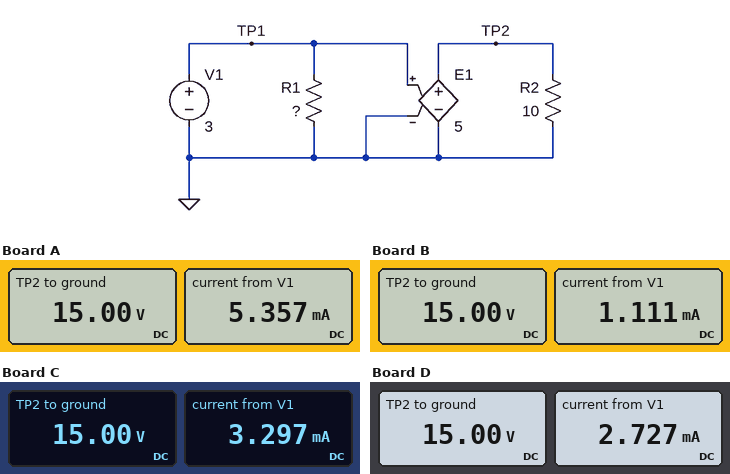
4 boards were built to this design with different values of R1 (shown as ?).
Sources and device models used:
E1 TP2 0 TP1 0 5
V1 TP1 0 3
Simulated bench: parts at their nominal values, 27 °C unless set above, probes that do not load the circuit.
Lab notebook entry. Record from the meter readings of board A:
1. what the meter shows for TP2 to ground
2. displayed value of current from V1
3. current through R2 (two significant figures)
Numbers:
15.00 V
5.357 mA
1.5 A
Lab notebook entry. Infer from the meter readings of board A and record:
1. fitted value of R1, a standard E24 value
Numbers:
560 Ω
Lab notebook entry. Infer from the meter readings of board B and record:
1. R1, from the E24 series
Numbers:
2.7 kΩ
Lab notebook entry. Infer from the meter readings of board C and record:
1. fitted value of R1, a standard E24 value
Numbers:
910 Ω
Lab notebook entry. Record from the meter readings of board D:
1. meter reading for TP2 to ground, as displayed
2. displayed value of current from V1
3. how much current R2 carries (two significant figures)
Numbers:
15.00 V
2.727 mA
1.5 A
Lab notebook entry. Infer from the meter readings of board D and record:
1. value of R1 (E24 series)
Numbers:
1.1 kΩ
